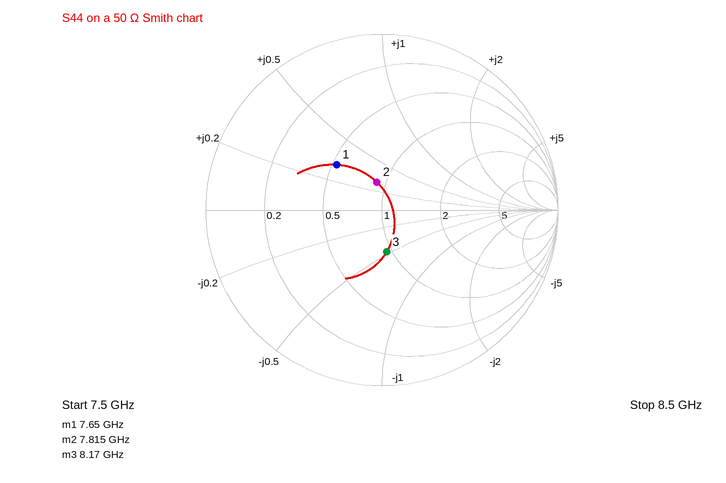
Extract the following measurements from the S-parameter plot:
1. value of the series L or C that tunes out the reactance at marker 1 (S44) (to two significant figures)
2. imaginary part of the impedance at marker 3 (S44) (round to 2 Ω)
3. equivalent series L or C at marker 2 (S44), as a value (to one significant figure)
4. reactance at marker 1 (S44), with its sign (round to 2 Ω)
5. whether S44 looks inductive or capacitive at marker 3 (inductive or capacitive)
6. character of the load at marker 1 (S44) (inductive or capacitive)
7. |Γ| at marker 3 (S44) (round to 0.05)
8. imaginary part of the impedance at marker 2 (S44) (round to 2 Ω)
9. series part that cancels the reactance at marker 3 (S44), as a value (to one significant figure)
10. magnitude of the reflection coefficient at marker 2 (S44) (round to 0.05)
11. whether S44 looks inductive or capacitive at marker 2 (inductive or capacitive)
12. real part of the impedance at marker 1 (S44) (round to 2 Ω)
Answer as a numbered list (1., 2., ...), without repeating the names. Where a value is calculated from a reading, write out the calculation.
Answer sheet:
1. C = 1/(2π × 7.65 GHz × 16 Ω) ≈ 1.3 pF
2. -24 Ω
3. L = 14 Ω/(2π × 7.815 GHz) ≈ 285 pH, so 300 pH to one significant figure
4. +16 Ω
5. capacitive
6. inductive
7. 0.25
8. +14 Ω
9. L = 24 Ω/(2π × 8.17 GHz) ≈ 468 pH, so 500 pH to one significant figure
10. 0.15
11. inductive
12. 26 Ω
